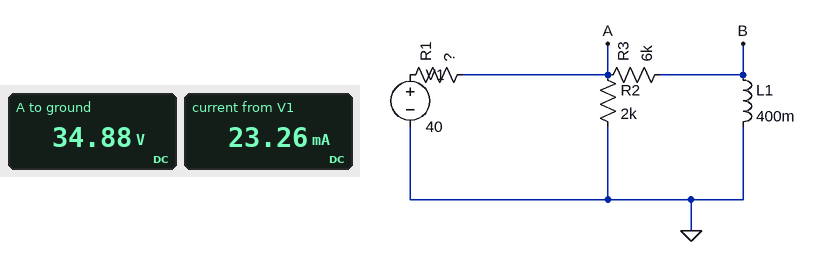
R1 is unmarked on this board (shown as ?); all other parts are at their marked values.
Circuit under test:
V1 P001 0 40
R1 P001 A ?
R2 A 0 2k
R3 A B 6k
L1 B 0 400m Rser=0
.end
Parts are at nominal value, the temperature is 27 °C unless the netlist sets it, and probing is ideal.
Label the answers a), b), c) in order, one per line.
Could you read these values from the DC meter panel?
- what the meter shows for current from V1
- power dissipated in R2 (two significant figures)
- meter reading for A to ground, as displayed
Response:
a) 23.26 mA
b) 610 mW
c) 34.88 V
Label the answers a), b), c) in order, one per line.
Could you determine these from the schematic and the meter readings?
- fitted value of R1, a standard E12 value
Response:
a) 220 Ω
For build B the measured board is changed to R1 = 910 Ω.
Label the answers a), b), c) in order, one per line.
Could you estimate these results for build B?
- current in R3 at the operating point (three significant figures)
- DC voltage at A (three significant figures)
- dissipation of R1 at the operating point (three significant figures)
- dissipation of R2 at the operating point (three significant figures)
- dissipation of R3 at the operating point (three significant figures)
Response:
a) 4.15 mA
b) 24.9 V
c) 251 mW
d) 310 mW
e) 103 mW
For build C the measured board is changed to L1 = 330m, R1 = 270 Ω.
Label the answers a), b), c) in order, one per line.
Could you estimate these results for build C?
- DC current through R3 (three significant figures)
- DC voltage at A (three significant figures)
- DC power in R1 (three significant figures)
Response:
a) 5.65 mA
b) 33.9 V
c) 138 mW
